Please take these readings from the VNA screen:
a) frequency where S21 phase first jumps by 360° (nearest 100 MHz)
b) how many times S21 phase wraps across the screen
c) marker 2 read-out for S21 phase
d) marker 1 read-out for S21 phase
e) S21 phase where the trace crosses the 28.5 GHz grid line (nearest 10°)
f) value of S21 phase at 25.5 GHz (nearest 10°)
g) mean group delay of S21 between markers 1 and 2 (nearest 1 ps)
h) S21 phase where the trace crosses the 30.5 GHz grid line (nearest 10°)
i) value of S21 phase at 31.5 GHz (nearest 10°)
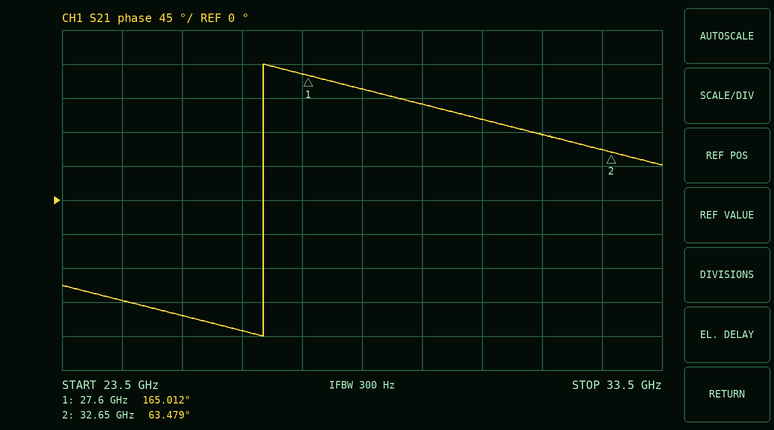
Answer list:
26.9 GHz
1
63.479°
165.012°
150°
-150°
56 ps
110°
90°
